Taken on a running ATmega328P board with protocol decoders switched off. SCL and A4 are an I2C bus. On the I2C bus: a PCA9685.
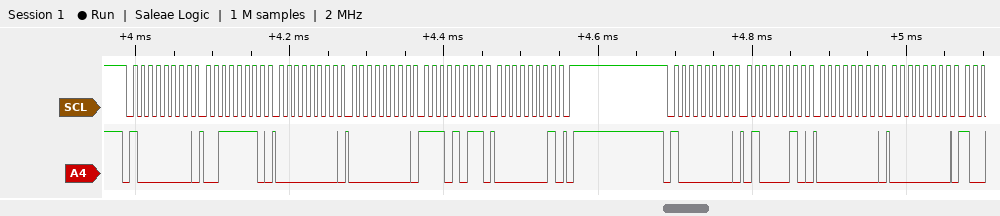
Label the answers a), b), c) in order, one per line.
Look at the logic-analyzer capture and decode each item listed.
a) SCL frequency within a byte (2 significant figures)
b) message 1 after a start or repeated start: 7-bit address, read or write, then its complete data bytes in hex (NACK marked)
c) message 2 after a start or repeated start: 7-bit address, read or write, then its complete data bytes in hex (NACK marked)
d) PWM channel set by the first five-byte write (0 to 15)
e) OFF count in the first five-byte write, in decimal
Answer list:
a) 100 kHz
b) 0x40 write: 3E 00 00 EB 01
c) 0x40 write: 42 00 00
d) 14
e) 491
